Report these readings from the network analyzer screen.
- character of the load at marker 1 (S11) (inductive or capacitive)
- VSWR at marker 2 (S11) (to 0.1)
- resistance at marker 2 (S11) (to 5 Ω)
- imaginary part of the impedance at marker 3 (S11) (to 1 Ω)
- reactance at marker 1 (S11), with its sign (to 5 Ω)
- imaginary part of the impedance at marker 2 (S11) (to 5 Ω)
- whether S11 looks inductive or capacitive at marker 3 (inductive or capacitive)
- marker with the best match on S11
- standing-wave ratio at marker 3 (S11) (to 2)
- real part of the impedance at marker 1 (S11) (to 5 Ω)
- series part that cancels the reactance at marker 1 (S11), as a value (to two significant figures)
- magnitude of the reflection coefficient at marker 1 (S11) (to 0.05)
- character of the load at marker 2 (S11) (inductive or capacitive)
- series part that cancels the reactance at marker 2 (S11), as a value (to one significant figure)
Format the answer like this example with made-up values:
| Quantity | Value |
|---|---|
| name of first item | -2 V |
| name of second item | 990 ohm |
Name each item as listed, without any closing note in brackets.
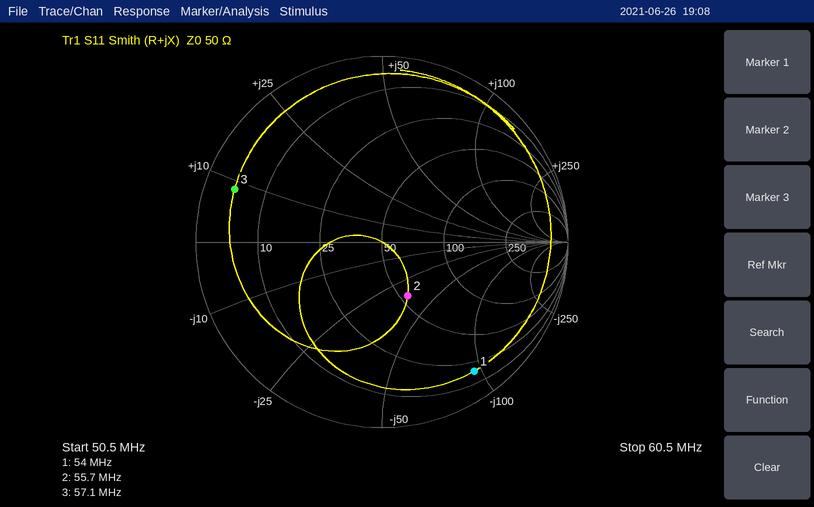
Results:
| Quantity | Value |
|---|---|
| character of the load at marker 1 (S11) | capacitive |
| VSWR at marker 2 (S11) | 1.9 |
| resistance at marker 2 (S11) | 55 Ω |
| imaginary part of the impedance at marker 3 (S11) | +9 Ω |
| reactance at marker 1 (S11), with its sign | -95 Ω |
| imaginary part of the impedance at marker 2 (S11) | -35 Ω |
| whether S11 looks inductive or capacitive at marker 3 | inductive |
| marker with the best match on S11 | marker 2 |
| standing-wave ratio at marker 3 (S11) | 12 |
| real part of the impedance at marker 1 (S11) | 20 Ω |
| series part that cancels the reactance at marker 1 (S11), as a value | 280 nH |
| magnitude of the reflection coefficient at marker 1 (S11) | 0.85 |
| character of the load at marker 2 (S11) | capacitive |
| series part that cancels the reactance at marker 2 (S11), as a value | 100 nH |
